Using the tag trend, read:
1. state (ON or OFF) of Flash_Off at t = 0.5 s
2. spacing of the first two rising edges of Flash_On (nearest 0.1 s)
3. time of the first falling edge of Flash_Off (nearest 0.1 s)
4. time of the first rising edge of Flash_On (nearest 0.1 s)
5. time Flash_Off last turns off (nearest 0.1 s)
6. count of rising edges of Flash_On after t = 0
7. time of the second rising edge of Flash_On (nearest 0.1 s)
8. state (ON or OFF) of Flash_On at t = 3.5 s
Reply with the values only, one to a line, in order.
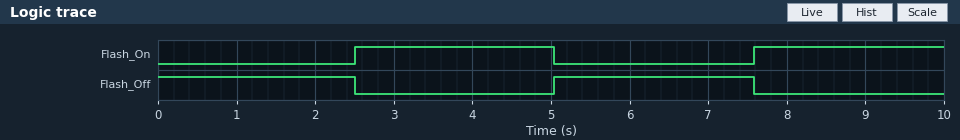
ON
5.1 s
2.5 s
2.5 s
7.6 s
2
7.6 s
ON
